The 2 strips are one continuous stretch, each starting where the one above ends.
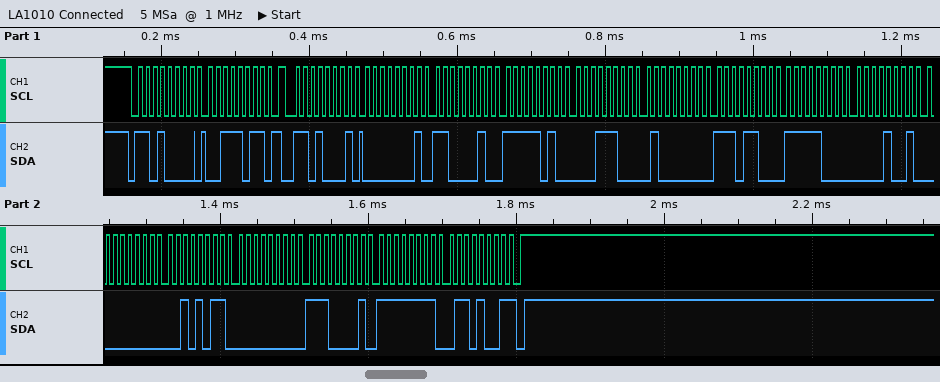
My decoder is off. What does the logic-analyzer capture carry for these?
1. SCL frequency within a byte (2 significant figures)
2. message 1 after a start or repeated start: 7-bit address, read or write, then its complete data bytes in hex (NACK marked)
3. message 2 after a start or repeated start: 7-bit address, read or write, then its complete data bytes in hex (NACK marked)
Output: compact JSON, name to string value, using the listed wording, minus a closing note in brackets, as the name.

{"SCL frequency within a byte": "100 kHz", "message 1 after a start or repeated start: 7-bit address, read or write, then its complete data bytes in hex": "0x68 write: 3B", "message 2 after a start or repeated start: 7-bit address, read or write, then its complete data bytes in hex": "0x68 read: 01 C2 FA 1C 40 EC F8 09 00 2B 00 E1 FF 69 NACK"}
